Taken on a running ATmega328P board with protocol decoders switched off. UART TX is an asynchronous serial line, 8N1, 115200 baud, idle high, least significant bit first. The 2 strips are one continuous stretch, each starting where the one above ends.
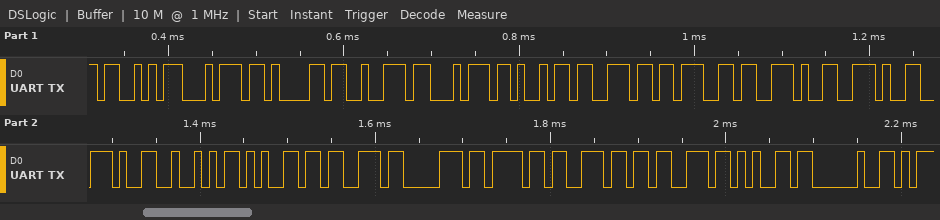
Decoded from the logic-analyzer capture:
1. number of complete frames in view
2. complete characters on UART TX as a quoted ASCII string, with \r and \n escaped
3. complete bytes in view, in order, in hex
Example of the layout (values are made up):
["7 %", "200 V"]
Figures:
["20", "\"Starting...Response \"", "0x53 0x74 0x61 0x72 0x74 0x69 0x6E 0x67 0x2E 0x2E 0x2E 0x52 0x65 0x73 0x70 0x6F 0x6E 0x73 0x65 0x20"]
